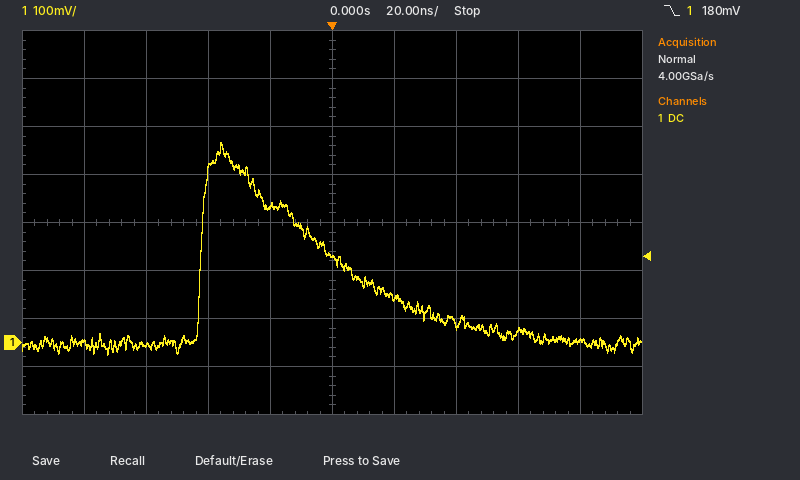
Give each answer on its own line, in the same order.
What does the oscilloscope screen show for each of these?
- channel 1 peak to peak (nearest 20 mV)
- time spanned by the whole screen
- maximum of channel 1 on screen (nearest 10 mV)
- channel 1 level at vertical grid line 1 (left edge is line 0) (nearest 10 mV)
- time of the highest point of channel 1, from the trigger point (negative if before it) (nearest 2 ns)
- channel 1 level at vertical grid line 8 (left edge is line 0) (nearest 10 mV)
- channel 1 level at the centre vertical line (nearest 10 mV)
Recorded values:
440 mV
200 ns
420 mV
0 mV
-36 ns
20 mV
180 mV
